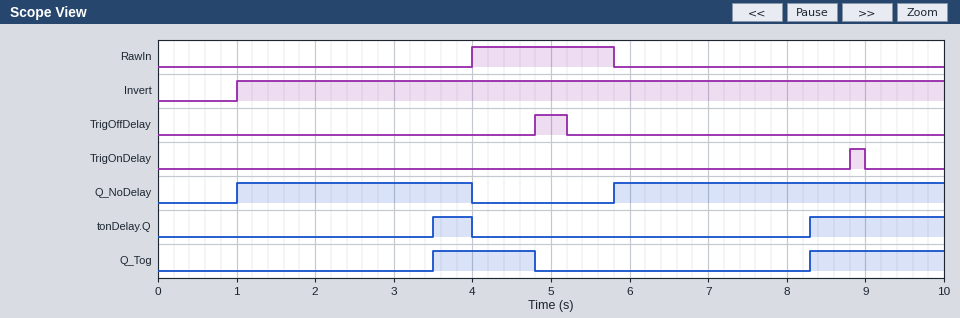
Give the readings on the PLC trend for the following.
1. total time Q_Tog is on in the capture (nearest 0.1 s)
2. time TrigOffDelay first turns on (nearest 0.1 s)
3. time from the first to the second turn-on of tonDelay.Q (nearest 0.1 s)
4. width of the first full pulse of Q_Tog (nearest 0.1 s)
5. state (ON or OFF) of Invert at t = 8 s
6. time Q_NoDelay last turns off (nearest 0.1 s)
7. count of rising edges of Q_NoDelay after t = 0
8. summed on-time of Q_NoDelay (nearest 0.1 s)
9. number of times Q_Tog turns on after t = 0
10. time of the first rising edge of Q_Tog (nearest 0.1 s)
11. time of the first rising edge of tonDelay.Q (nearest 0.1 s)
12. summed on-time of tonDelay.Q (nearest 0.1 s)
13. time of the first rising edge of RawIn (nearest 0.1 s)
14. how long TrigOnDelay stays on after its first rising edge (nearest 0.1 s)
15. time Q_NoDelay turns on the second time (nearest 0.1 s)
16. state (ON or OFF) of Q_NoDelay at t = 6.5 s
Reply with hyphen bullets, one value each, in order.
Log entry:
- 3.0 s
- 4.8 s
- 4.8 s
- 1.3 s
- ON
- 4.0 s
- 2
- 7.2 s
- 2
- 3.5 s
- 3.5 s
- 2.2 s
- 4.0 s
- 0.2 s
- 5.8 s
- ON
